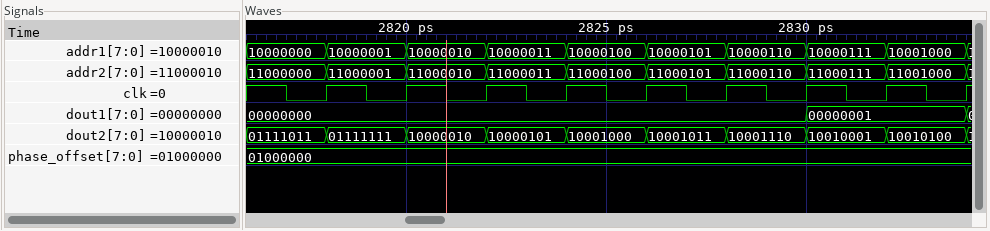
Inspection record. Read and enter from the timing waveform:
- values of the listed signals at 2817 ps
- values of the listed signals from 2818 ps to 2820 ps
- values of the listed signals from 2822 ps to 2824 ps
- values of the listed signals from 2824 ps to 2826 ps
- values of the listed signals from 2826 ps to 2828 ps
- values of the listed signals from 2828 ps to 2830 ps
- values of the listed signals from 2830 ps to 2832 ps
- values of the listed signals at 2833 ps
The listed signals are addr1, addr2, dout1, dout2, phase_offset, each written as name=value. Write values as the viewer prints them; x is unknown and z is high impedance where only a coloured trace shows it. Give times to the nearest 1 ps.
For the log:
addr1=10000000, addr2=11000000, dout1=00000000, dout2=01111011, phase_offset=01000000
addr1=10000001, addr2=11000001, dout1=00000000, dout2=01111111, phase_offset=01000000
addr1=10000011, addr2=11000011, dout1=00000000, dout2=10000101, phase_offset=01000000
addr1=10000100, addr2=11000100, dout1=00000000, dout2=10001000, phase_offset=01000000
addr1=10000101, addr2=11000101, dout1=00000000, dout2=10001011, phase_offset=01000000
addr1=10000110, addr2=11000110, dout1=00000000, dout2=10001110, phase_offset=01000000
addr1=10000111, addr2=11000111, dout1=00000001, dout2=10010001, phase_offset=01000000
addr1=10001000, addr2=11001000, dout1=00000001, dout2=10010100, phase_offset=01000000
